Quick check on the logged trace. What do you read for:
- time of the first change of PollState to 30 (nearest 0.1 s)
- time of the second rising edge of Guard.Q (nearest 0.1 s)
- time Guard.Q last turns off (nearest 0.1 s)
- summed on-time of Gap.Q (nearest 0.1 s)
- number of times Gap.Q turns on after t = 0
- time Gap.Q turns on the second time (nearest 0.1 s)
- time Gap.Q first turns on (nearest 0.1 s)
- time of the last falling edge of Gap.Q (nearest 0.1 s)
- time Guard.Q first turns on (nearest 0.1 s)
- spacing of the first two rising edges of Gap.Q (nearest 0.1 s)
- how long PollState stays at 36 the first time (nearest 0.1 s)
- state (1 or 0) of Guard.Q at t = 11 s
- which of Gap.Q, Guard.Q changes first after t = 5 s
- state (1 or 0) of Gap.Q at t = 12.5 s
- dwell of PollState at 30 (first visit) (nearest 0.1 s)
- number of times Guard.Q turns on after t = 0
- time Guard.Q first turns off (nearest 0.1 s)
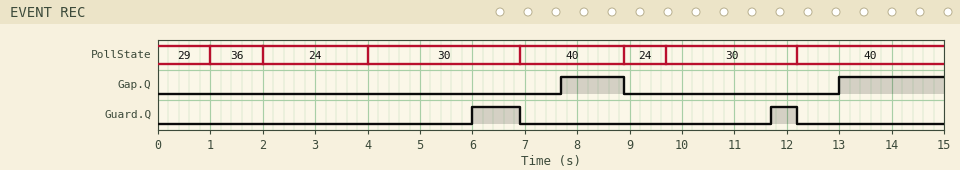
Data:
4.0 s
11.7 s
12.2 s
3.2 s
2
13.0 s
7.7 s
8.9 s
6.0 s
5.3 s
1.0 s
0
Guard.Q
0
2.9 s
2
6.9 s
